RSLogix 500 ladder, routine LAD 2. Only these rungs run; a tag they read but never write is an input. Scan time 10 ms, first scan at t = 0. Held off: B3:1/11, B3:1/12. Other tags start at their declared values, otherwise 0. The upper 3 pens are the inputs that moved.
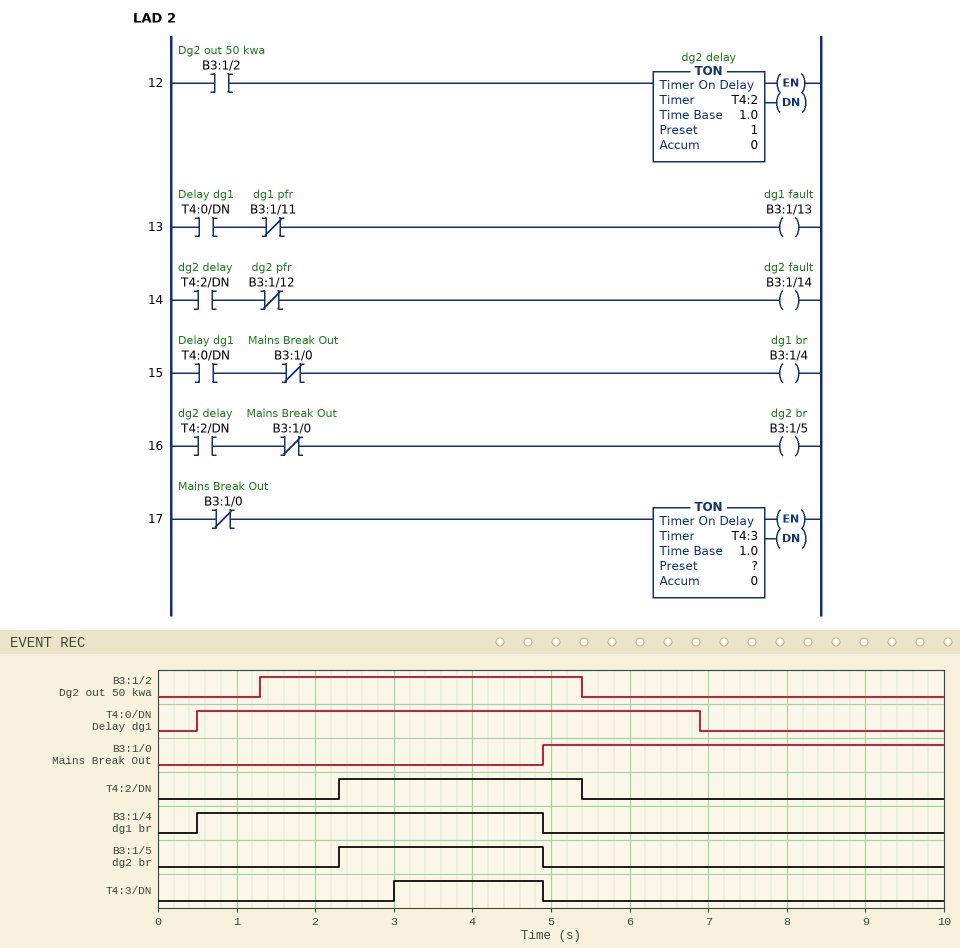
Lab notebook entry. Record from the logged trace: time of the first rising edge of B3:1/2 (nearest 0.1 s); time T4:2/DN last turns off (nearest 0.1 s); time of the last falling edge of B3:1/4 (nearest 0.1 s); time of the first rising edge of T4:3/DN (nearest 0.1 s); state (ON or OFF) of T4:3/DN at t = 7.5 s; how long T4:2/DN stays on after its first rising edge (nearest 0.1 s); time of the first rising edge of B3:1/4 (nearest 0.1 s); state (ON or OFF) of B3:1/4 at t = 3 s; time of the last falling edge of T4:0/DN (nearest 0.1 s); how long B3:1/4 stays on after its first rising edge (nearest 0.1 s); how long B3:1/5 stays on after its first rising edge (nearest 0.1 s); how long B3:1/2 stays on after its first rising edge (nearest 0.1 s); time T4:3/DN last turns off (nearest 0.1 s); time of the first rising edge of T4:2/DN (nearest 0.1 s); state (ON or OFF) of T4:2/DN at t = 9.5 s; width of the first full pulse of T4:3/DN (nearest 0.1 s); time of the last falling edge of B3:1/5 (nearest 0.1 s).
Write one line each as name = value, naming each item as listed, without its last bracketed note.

time of the first rising edge of B3:1/2 = 1.3 s
time T4:2/DN last turns off = 5.4 s
time of the last falling edge of B3:1/4 = 4.9 s
time of the first rising edge of T4:3/DN = 3.0 s
state (ON or OFF) of T4:3/DN at t = 7.5 s = OFF
how long T4:2/DN stays on after its first rising edge = 3.1 s
time of the first rising edge of B3:1/4 = 0.5 s
state (ON or OFF) of B3:1/4 at t = 3 s = ON
time of the last falling edge of T4:0/DN = 6.9 s
how long B3:1/4 stays on after its first rising edge = 4.4 s
how long B3:1/5 stays on after its first rising edge = 2.6 s
how long B3:1/2 stays on after its first rising edge = 4.1 s
time T4:3/DN last turns off = 4.9 s
time of the first rising edge of T4:2/DN = 2.3 s
state (ON or OFF) of T4:2/DN at t = 9.5 s = OFF
width of the first full pulse of T4:3/DN = 1.9 s
time of the last falling edge of B3:1/5 = 4.9 s
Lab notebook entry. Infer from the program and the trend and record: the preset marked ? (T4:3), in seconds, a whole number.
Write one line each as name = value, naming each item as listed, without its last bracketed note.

the preset marked ? (T4:3), in seconds, a whole number = 3 s
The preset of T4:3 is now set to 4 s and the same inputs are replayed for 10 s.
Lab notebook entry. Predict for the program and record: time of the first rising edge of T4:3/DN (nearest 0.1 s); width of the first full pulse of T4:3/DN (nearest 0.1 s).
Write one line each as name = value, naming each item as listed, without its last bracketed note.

time of the first rising edge of T4:3/DN = 4.0 s
width of the first full pulse of T4:3/DN = 0.9 s
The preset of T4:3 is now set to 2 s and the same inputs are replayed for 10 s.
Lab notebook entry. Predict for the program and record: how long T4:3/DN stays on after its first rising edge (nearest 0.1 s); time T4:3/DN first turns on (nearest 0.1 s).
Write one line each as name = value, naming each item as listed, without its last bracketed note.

how long T4:3/DN stays on after its first rising edge = 2.9 s
time T4:3/DN first turns on = 2.0 s
